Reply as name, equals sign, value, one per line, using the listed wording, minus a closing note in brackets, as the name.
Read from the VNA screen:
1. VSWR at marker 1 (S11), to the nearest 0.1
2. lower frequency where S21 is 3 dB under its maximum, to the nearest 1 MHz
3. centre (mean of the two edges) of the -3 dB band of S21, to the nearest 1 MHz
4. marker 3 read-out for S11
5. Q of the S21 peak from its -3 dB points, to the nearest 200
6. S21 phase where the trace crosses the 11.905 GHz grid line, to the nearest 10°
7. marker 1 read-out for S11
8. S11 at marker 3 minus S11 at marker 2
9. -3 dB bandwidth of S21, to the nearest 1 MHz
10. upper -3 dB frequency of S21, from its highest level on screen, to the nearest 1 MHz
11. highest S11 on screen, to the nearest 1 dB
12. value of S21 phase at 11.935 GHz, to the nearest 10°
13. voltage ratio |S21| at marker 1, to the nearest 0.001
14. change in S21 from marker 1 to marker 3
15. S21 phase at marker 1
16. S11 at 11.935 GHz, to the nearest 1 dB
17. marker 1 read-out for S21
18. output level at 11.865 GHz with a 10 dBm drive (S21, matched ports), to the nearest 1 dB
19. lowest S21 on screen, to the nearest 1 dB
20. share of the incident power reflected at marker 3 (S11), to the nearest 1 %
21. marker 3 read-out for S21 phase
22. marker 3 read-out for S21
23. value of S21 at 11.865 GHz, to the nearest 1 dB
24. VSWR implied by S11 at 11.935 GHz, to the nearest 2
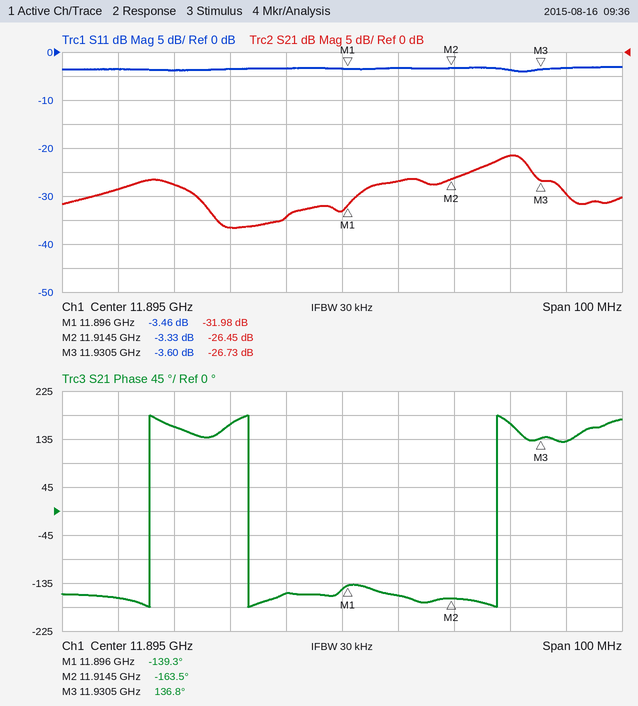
VSWR at marker 1 (S11), to the nearest 0.1 = 5.1
lower frequency where S21 is 3 dB under its maximum, to the nearest 1 MHz = 11.919 GHz
centre (mean of the two edges) of the -3 dB band of S21, to the nearest 1 MHz = 11.924 GHz
marker 3 read-out for S11 = -3.60 dB
Q of the S21 peak from its -3 dB points, to the nearest 200 = 1200
S21 phase where the trace crosses the 11.905 GHz grid line, to the nearest 10° = -160°
marker 1 read-out for S11 = -3.46 dB
S11 at marker 3 minus S11 at marker 2 = -0.27 dB
-3 dB bandwidth of S21, to the nearest 1 MHz = 10 MHz
upper -3 dB frequency of S21, from its highest level on screen, to the nearest 1 MHz = 11.929 GHz
highest S11 on screen, to the nearest 1 dB = -3 dB
value of S21 phase at 11.935 GHz, to the nearest 10° = 130°
voltage ratio |S21| at marker 1, to the nearest 0.001 = 0.025
change in S21 from marker 1 to marker 3 = 5.25 dB
S21 phase at marker 1 = -139.3°
S11 at 11.935 GHz, to the nearest 1 dB = -3 dB
marker 1 read-out for S21 = -31.98 dB
output level at 11.865 GHz with a 10 dBm drive (S21, matched ports), to the nearest 1 dB = -18 dBm
lowest S21 on screen, to the nearest 1 dB = -37 dB
share of the incident power reflected at marker 3 (S11), to the nearest 1 % = 44 %
marker 3 read-out for S21 phase = 136.8°
marker 3 read-out for S21 = -26.73 dB
value of S21 at 11.865 GHz, to the nearest 1 dB = -28 dB
VSWR implied by S11 at 11.935 GHz, to the nearest 2 = 6
